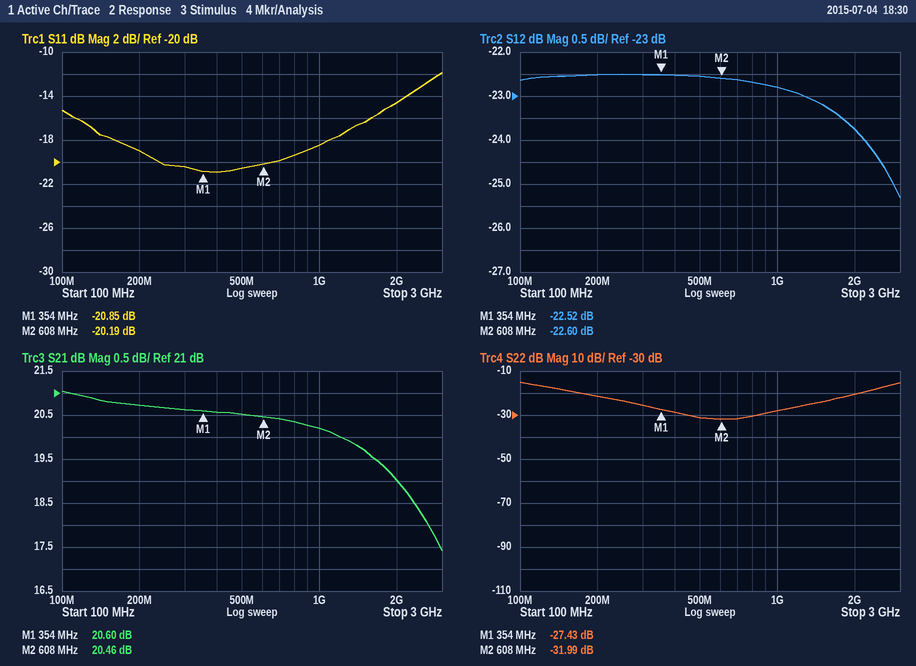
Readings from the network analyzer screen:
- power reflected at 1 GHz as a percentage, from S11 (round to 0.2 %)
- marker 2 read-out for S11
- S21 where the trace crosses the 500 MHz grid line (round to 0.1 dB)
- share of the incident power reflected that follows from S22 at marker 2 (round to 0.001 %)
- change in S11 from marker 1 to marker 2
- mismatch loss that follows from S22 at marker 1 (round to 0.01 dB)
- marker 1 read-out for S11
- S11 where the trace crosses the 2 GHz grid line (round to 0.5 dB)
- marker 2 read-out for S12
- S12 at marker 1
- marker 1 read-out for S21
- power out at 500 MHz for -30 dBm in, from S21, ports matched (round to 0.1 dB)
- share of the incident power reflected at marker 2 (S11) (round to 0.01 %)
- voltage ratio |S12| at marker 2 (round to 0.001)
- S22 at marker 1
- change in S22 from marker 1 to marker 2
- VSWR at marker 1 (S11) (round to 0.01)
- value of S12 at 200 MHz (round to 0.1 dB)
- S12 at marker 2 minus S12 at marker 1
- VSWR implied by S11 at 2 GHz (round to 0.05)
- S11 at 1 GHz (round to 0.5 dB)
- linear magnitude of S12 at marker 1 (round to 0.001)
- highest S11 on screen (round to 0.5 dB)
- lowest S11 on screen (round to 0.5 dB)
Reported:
1.4 %
-20.19 dB
20.5 dB
0.063 %
0.66 dB
0.01 dB
-20.85 dB
-14.5 dB
-22.60 dB
-22.52 dB
20.60 dB
-9.5 dBm
0.96 %
0.074
-27.43 dB
-4.56 dB
1.20
-22.5 dB
-0.08 dB
1.45
-18.5 dB
0.075
-12.0 dB
-21.0 dB
